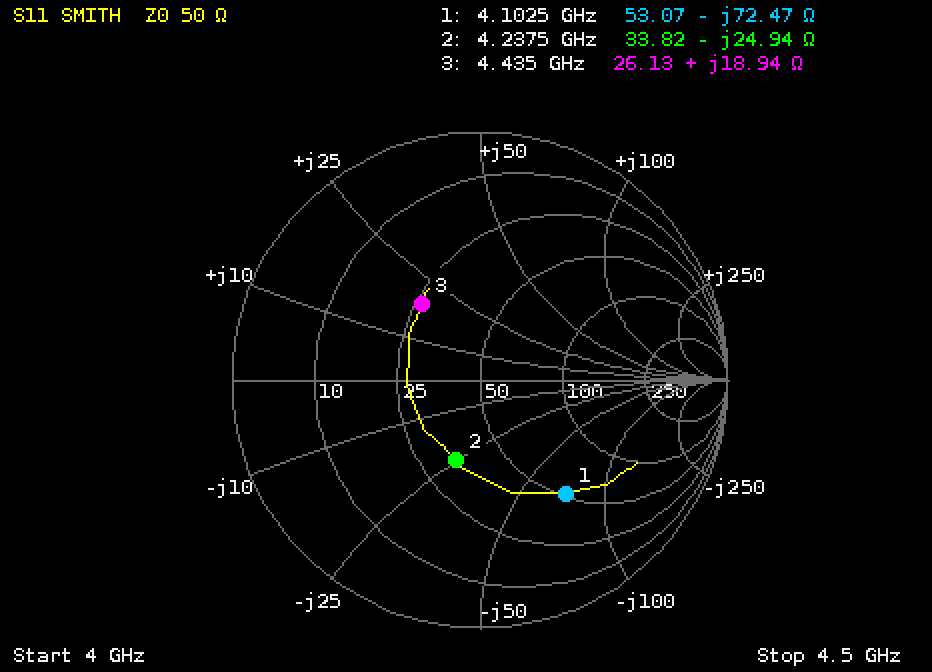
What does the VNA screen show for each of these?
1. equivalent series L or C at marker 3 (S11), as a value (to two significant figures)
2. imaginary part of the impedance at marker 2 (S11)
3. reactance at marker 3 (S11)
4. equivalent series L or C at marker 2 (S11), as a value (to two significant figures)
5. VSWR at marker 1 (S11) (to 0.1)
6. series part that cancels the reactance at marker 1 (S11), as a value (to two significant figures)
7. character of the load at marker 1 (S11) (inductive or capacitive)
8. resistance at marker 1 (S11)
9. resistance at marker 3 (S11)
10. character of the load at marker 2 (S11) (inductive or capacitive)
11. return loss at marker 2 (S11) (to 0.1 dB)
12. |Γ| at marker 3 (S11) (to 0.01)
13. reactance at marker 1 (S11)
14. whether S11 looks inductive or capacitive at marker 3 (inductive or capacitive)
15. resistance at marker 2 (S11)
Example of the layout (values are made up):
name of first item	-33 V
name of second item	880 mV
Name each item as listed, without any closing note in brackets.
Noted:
equivalent series L or C at marker 3 (S11), as a value	680 pH
imaginary part of the impedance at marker 2	-24.94 Ω
reactance at marker 3	+18.94 Ω
equivalent series L or C at marker 2 (S11), as a value	1.5 pF
VSWR at marker 1 (S11)	3.7
series part that cancels the reactance at marker 1 (S11), as a value	2.8 nH
character of the load at marker 1 (S11)	capacitive
resistance at marker 1	53.07 Ω
resistance at marker 3	26.13 Ω
character of the load at marker 2 (S11)	capacitive
return loss at marker 2 (S11)	9.4 dB
|Γ| at marker 3 (S11)	0.39
reactance at marker 1	-72.47 Ω
whether S11 looks inductive or capacitive at marker 3	inductive
resistance at marker 2	33.82 Ω
